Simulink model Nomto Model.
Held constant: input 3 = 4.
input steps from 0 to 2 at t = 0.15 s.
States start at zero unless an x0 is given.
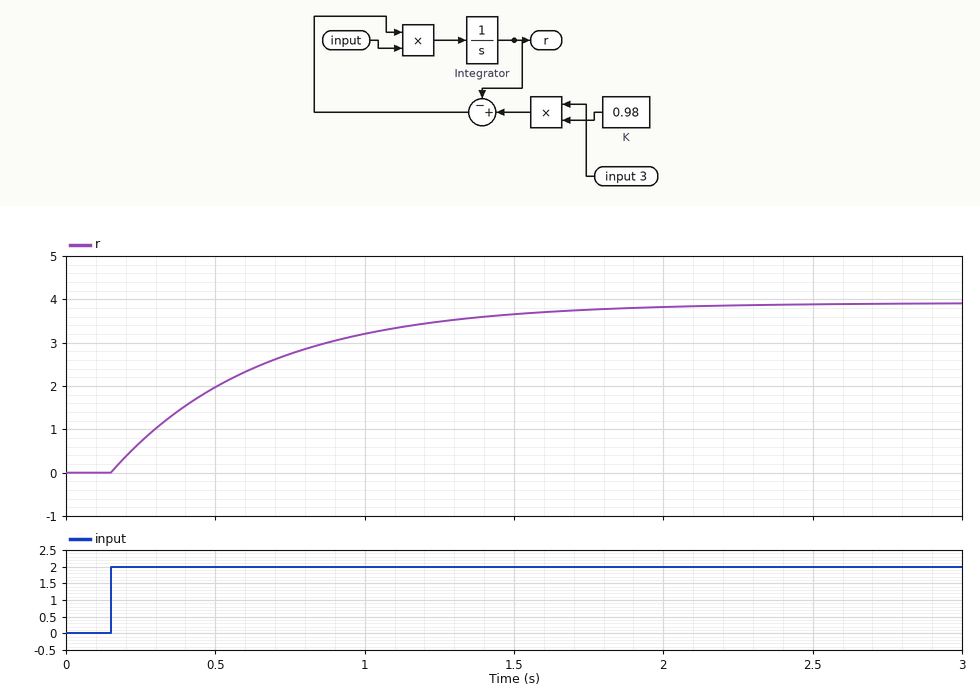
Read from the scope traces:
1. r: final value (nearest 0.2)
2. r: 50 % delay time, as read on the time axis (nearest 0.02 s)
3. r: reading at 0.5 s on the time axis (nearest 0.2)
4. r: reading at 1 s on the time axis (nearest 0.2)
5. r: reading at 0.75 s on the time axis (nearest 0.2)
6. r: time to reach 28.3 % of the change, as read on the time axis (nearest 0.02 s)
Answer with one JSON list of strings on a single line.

["4.0", "0.50 s", "2.0", "3.2", "2.8", "0.32 s"]
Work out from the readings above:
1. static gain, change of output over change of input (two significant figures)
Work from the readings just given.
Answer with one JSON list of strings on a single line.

["2.0"]
